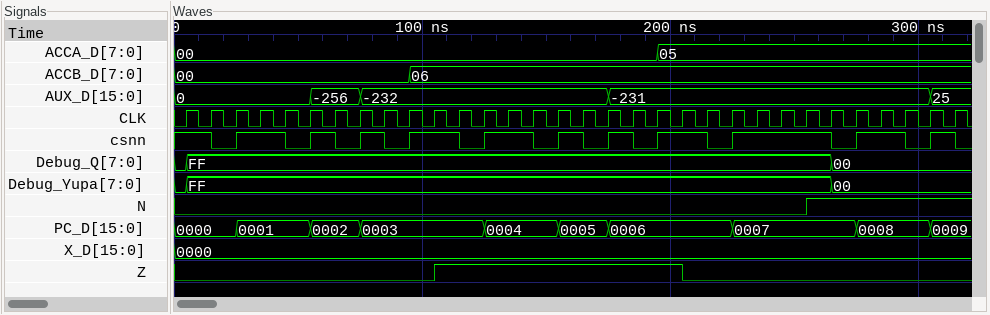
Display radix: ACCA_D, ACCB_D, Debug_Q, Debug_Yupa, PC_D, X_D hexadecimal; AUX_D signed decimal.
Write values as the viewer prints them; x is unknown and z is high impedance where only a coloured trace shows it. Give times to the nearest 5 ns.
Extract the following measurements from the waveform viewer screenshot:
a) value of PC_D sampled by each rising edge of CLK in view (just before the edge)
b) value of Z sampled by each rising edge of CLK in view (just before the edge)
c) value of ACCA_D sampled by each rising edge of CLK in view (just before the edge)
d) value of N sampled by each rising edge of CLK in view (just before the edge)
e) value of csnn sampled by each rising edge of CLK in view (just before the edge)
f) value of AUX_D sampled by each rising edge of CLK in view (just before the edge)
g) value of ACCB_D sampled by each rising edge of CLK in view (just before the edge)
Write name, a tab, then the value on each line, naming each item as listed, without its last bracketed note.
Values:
value of PC_D sampled by each rising edge of CLK in view	0000, 0000, 0000, 0001, 0001, 0001, 0002, 0002, 0003, 0003, 0003, 0003, 0003, 0004, 0004, 0004, 0005, 0005, 0006, 0006, 0006, 0006, 0006, 0007, 0007, 0007, 0007, 0007, 0008, 0008, 0008, 0009
value of Z sampled by each rising edge of CLK in view	0 0 0 0 0 0 0 0 0 0 0 1 1 1 1 1 1 1 1 1 1 0 0 0 0 0 0 0 0 0 0 0
value of ACCA_D sampled by each rising edge of CLK in view	00, 00, 00, 00, 00, 00, 00, 00, 00, 00, 00, 00, 00, 00, 00, 00, 00, 00, 00, 00, 05, 05, 05, 05, 05, 05, 05, 05, 05, 05, 05, 05
value of N sampled by each rising edge of CLK in view	0 0 0 0 0 0 0 0 0 0 0 0 0 0 0 0 0 0 0 0 0 0 0 0 0 0 1 1 1 1 1 1
value of csnn sampled by each rising edge of CLK in view	1 1 0 1 1 0 1 0 1 0 1 1 0 1 1 0 1 0 1 0 1 1 0 1 1 1 1 0 1 1 0 1
value of AUX_D sampled by each rising edge of CLK in view	0, 0, 0, 0, 0, 0, -256, -256, -232, -232, -232, -232, -232, -232, -232, -232, -232, -232, -231, -231, -231, -231, -231, -231, -231, -231, -231, -231, -231, -231, -231, 25
value of ACCB_D sampled by each rising edge of CLK in view	00, 00, 00, 00, 00, 00, 00, 00, 00, 00, 06, 06, 06, 06, 06, 06, 06, 06, 06, 06, 06, 06, 06, 06, 06, 06, 06, 06, 06, 06, 06, 06
